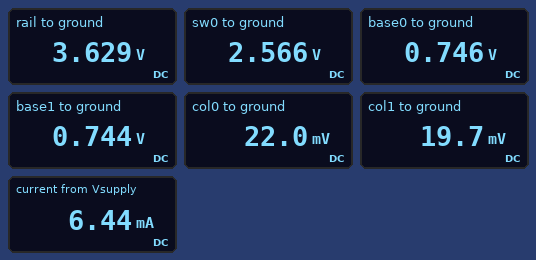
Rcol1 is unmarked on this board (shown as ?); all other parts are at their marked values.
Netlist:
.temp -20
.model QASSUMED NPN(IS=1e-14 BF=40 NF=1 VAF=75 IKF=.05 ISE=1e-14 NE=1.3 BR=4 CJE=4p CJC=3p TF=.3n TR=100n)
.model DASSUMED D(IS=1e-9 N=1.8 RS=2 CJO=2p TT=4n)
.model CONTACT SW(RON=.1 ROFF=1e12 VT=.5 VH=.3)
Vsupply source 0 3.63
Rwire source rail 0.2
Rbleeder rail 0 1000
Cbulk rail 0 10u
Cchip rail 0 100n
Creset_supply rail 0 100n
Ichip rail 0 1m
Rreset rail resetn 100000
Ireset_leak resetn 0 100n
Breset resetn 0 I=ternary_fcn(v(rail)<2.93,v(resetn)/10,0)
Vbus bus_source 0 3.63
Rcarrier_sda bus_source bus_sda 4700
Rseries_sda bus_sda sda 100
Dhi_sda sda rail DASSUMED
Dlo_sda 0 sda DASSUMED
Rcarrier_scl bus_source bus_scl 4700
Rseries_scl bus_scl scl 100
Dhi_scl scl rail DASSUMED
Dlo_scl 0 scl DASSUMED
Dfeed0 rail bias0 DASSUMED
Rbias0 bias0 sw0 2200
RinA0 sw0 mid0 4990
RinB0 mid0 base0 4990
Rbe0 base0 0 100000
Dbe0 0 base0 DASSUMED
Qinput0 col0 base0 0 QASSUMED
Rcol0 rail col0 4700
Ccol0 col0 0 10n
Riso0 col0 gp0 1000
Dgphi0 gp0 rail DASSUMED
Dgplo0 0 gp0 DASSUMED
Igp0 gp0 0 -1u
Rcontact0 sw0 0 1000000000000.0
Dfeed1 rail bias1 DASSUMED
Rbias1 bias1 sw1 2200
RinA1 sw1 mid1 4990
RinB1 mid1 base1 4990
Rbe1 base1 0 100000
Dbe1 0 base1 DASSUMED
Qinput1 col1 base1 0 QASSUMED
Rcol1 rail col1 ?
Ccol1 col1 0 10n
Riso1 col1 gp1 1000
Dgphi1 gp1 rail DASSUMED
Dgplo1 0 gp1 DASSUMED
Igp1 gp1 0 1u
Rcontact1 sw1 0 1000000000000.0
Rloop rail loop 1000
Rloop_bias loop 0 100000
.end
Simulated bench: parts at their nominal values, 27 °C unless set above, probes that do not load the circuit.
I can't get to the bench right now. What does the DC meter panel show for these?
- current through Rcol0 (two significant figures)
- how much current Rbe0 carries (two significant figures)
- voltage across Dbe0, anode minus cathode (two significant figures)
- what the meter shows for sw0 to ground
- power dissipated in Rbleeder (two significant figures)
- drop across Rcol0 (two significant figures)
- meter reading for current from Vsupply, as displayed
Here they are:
770 µA
7.5 µA
-750 mV
2.566 V
13 mW
3.6 V
6.44 mA
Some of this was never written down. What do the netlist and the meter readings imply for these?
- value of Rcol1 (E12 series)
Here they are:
5.6 kΩ
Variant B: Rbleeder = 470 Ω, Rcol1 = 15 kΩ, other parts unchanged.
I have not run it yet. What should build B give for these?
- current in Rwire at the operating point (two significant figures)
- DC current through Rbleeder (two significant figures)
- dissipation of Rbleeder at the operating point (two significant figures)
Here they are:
10 mA
7.7 mA
28 mW
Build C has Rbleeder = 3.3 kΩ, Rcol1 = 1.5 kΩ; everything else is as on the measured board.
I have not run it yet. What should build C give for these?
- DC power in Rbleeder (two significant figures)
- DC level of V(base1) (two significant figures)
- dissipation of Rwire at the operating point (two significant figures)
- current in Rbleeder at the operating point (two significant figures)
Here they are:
4.0 mW
760 mV
6.4 µW
1.1 mA
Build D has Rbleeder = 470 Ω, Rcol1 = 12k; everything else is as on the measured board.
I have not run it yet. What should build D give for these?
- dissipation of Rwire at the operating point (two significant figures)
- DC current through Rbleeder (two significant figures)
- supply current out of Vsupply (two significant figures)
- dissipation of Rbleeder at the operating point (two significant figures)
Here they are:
21 µW
7.7 mA
10 mA
28 mW
